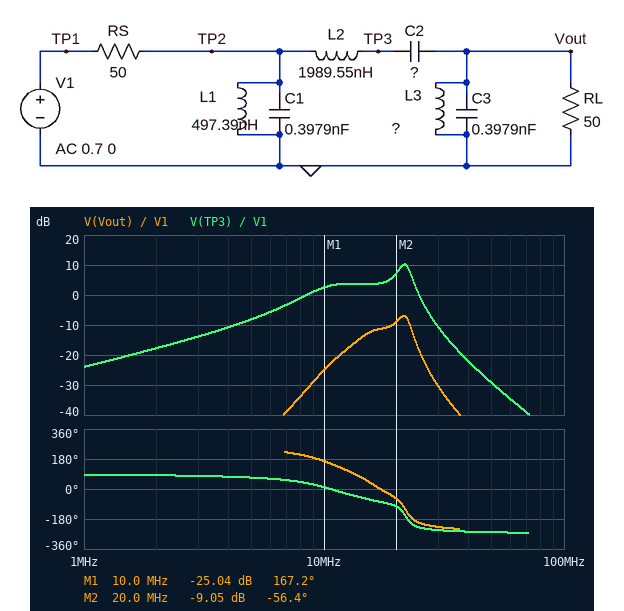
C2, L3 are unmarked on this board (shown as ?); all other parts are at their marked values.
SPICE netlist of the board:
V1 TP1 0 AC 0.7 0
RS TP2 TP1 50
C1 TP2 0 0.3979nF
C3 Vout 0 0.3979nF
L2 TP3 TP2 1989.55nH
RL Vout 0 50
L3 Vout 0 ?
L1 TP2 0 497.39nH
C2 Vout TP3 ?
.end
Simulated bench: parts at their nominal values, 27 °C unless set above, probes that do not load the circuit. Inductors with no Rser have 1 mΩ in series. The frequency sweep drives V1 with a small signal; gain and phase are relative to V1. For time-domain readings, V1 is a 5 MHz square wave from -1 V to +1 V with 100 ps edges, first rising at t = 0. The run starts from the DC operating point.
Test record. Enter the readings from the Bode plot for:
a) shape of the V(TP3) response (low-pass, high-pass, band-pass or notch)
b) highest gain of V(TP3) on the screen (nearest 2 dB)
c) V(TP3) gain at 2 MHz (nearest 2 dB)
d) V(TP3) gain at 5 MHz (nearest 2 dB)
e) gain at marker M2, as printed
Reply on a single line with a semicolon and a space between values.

band-pass; 10 dB; -18 dB; -8 dB; -9.05 dB
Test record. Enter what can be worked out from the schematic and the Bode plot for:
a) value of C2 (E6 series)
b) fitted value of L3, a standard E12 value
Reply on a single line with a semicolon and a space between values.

33 pF; 220 nH
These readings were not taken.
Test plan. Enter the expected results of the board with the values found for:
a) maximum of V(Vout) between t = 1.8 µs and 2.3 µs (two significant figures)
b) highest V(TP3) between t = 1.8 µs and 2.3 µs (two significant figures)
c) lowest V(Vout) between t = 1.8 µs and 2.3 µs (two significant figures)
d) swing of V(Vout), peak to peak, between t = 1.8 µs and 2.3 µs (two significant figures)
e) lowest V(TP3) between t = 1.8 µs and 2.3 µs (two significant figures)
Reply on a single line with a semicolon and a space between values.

120 mV; 1.2 V; -120 mV; 250 mV; -1.2 V
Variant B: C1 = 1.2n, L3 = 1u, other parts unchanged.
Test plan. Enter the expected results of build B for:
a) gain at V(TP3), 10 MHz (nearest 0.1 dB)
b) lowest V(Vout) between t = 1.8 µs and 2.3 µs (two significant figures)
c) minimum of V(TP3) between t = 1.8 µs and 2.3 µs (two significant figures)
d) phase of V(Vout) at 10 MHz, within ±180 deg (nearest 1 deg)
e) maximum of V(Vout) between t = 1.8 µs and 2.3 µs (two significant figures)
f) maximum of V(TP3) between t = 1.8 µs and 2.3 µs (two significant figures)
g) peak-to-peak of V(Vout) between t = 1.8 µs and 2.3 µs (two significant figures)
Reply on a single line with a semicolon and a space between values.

-5.5 dB; -51 mV; -1.0 V; -7 deg; 51 mV; 1.0 V; 100 mV
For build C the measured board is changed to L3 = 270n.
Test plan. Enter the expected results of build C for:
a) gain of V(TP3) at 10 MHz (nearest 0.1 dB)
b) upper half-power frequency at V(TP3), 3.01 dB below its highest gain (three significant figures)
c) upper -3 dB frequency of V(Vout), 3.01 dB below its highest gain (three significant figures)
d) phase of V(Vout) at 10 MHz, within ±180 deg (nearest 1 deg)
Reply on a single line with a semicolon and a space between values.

2.5 dB; 22.6 MHz; 22.5 MHz; 159 deg
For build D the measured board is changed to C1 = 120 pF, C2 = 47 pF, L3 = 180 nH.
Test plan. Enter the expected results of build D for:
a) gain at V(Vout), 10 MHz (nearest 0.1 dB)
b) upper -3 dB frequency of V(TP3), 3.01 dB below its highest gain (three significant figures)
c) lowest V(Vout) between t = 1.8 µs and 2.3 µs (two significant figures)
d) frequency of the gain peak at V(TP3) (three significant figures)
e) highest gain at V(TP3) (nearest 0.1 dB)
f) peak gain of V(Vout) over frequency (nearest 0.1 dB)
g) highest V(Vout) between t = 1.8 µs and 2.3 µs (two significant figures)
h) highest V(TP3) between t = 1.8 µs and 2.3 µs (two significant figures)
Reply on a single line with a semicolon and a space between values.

-25.4 dB; 15.8 MHz; -240 mV; 14.0 MHz; 10.3 dB; -6.4 dB; 240 mV; 1.9 V
